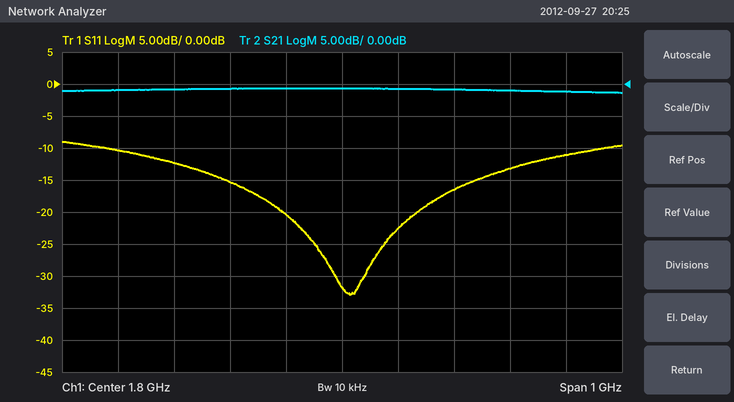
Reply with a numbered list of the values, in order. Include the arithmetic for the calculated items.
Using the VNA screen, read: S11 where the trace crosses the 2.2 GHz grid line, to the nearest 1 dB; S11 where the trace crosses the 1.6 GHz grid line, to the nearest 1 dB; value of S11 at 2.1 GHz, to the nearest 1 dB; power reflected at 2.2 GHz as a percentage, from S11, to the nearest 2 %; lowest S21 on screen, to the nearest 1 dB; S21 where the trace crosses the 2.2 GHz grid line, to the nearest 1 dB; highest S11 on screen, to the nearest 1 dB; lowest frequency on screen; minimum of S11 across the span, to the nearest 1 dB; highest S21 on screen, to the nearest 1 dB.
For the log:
1. -11 dB
2. -15 dB
3. -13 dB
4. 10^(-11/10) ≈ 8 %
5. -1 dB
6. -1 dB
7. -9 dB
8. 1.3 GHz
9. -33 dB
10. -1 dB
